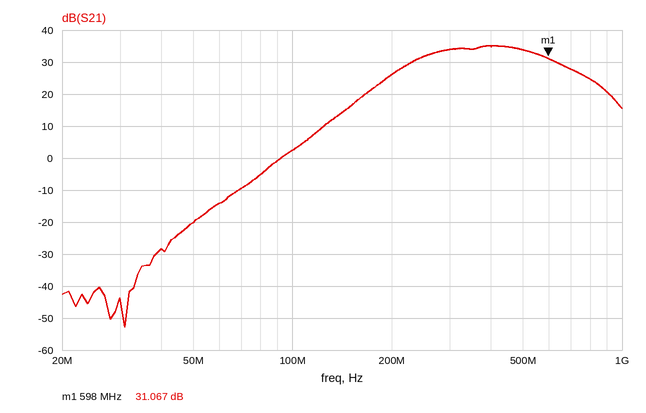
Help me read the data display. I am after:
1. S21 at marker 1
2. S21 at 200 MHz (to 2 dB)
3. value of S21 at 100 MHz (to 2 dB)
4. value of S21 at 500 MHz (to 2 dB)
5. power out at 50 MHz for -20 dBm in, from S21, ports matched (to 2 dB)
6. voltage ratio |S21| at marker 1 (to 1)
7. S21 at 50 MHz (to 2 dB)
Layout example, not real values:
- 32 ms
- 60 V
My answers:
- 31.067 dB
- 26 dB
- 2 dB
- 34 dB
- -40 dBm
- 36
- -20 dB
